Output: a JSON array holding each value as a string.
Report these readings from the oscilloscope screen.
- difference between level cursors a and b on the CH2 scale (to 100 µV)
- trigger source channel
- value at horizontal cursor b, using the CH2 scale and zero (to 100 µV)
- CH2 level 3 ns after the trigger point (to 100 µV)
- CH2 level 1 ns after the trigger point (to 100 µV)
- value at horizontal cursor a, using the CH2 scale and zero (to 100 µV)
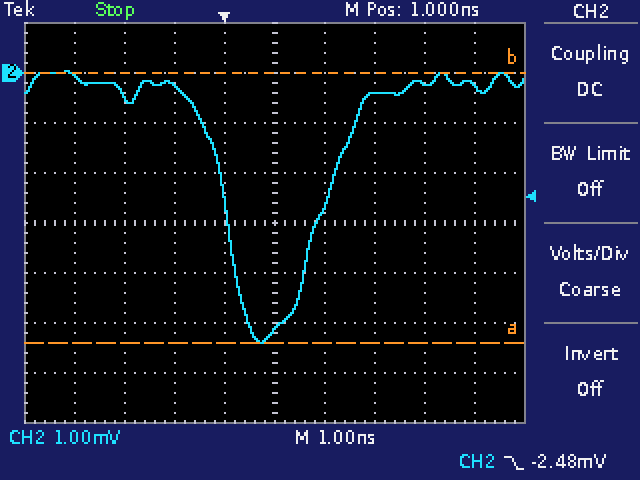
["5.4 mV", "CH2", "0.0 mV", "-400 µV", "-5.1 mV", "-5.4 mV"]
